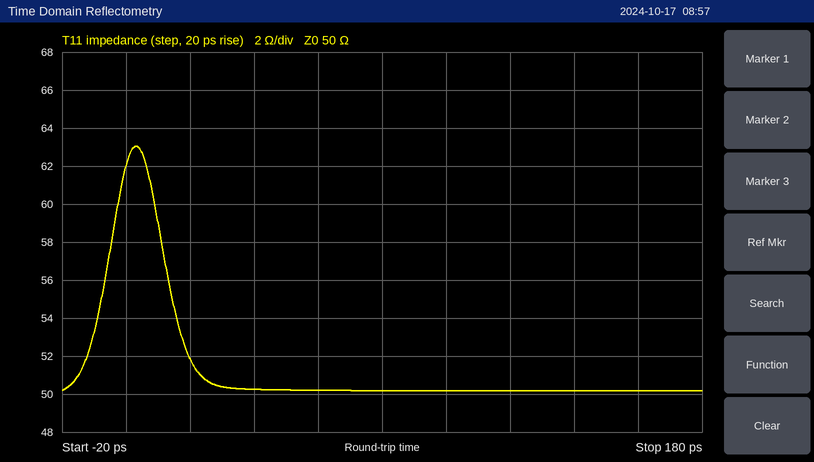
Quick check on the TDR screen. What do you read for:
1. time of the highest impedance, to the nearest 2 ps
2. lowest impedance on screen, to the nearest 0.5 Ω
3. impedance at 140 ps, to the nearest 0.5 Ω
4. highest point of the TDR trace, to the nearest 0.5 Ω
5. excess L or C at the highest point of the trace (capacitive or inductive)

4 ps
50.0 Ω
50.0 Ω
63.0 Ω
inductive
